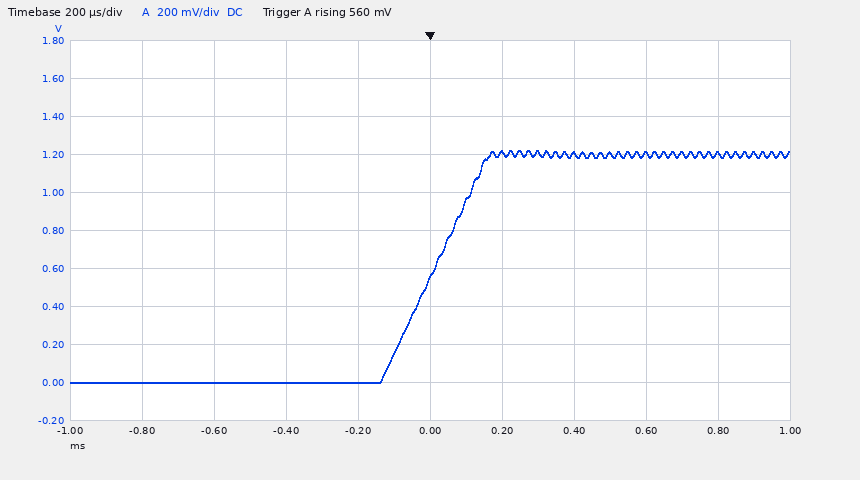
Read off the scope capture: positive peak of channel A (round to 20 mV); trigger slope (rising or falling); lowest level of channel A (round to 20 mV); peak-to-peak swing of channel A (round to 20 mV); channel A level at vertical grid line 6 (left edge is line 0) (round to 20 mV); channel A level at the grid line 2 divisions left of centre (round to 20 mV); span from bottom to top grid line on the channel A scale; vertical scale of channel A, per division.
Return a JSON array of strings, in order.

["1.22 V", "rising", "0 mV", "1.22 V", "1.20 V", "0 mV", "2 V", "200 mV"]
